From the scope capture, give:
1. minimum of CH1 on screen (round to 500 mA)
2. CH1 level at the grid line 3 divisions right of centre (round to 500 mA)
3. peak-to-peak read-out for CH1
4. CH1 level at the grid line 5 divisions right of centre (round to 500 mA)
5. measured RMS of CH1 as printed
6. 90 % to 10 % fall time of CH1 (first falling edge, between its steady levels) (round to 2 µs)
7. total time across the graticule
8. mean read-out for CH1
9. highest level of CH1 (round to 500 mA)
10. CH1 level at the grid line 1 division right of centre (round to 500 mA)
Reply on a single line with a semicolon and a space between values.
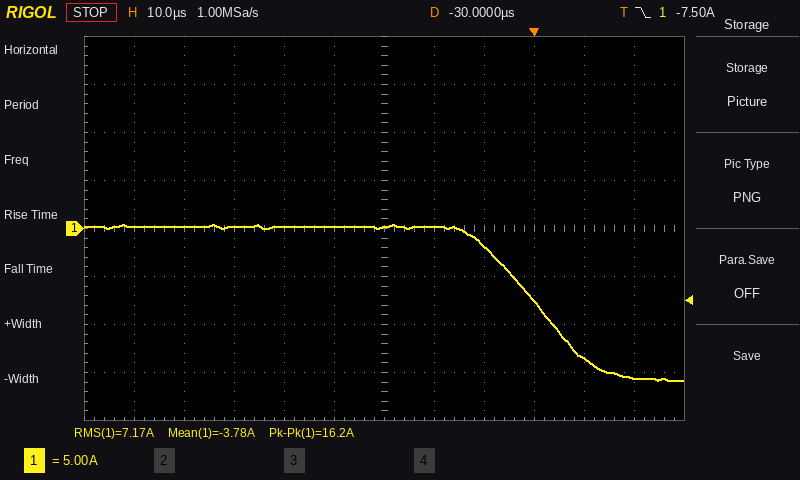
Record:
-16.0 A; -7.5 A; 16.2 A; -15.5 A; 7.17 A; 22 µs; 120 µs; -3.78 A; 500 mA; 0.0 A
